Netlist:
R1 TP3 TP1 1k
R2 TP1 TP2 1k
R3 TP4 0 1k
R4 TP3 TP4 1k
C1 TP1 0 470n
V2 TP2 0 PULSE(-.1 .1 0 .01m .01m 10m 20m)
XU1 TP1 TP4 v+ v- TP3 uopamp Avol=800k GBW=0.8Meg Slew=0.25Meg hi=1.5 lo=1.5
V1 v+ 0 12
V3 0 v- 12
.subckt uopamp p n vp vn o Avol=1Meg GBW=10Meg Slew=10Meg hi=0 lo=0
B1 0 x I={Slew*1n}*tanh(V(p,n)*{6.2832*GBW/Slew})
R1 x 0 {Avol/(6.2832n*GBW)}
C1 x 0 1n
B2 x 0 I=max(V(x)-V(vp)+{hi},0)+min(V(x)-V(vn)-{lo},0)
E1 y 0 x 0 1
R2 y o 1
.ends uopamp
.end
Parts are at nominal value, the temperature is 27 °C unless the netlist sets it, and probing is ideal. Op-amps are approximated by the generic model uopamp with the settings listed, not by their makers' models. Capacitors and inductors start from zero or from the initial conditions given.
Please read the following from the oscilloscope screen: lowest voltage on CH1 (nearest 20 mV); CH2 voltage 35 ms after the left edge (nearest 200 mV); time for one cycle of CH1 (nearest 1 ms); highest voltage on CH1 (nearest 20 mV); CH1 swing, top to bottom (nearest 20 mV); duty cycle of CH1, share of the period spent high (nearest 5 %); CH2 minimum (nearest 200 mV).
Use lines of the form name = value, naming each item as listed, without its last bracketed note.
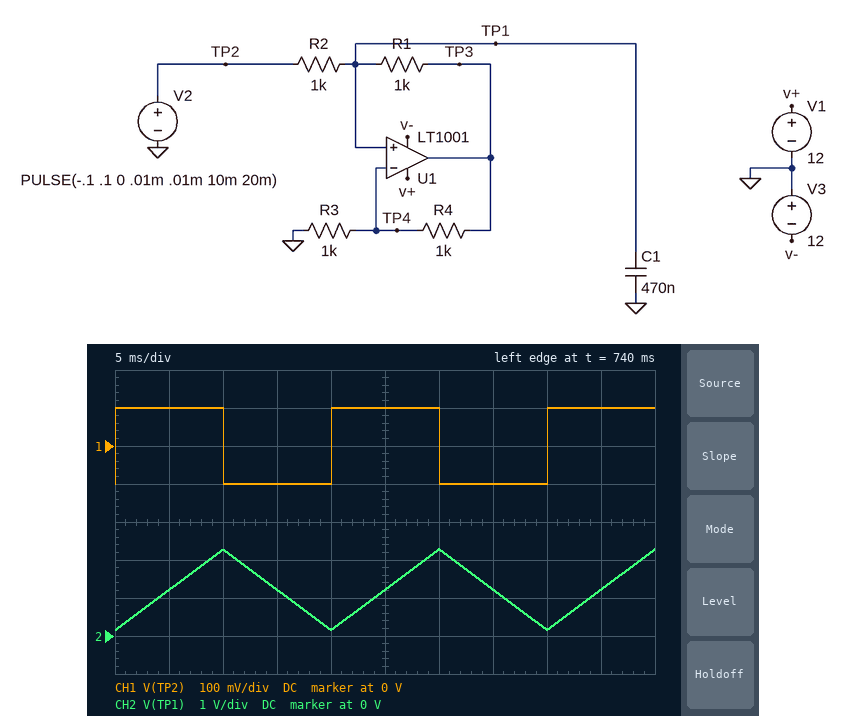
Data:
lowest voltage on CH1 = -100 mV
CH2 voltage 35 ms after the left edge = 1.2 V
time for one cycle of CH1 = 20 ms
highest voltage on CH1 = 100 mV
CH1 swing, top to bottom = 200 mV
duty cycle of CH1, share of the period spent high = 50 %
CH2 minimum = 200 mV
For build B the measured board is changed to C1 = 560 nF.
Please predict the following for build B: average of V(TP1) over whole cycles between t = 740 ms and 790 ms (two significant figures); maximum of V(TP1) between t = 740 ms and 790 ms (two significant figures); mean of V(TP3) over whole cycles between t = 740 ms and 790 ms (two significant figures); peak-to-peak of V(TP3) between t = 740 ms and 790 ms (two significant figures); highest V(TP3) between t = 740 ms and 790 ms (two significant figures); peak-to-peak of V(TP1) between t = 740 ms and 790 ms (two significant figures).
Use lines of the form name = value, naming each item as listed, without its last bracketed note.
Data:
average of V(TP1) over whole cycles between t = 740 ms and 790 ms = 1.0 V
maximum of V(TP1) between t = 740 ms and 790 ms = 1.9 V
mean of V(TP3) over whole cycles between t = 740 ms and 790 ms = 2.0 V
peak-to-peak of V(TP3) between t = 740 ms and 790 ms = 3.6 V
highest V(TP3) between t = 740 ms and 790 ms = 3.8 V
peak-to-peak of V(TP1) between t = 740 ms and 790 ms = 1.8 V
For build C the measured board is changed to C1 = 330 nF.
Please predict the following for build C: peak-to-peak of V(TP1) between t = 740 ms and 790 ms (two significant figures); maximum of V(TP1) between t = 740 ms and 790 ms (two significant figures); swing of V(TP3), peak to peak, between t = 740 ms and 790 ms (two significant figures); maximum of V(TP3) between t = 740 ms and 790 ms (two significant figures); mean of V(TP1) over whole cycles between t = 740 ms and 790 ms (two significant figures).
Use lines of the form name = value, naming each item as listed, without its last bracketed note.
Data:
peak-to-peak of V(TP1) between t = 740 ms and 790 ms = 3.0 V
maximum of V(TP1) between t = 740 ms and 790 ms = 3.2 V
swing of V(TP3), peak to peak, between t = 740 ms and 790 ms = 6.1 V
maximum of V(TP3) between t = 740 ms and 790 ms = 6.5 V
mean of V(TP1) over whole cycles between t = 740 ms and 790 ms = 1.7 V
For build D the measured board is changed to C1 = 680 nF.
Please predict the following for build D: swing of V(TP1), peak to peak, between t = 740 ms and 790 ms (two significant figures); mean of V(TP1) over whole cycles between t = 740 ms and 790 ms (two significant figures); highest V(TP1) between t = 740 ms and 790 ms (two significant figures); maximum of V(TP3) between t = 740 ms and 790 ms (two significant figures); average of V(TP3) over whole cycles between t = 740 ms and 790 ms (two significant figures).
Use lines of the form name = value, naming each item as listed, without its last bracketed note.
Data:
swing of V(TP1), peak to peak, between t = 740 ms and 790 ms = 1.5 V
mean of V(TP1) over whole cycles between t = 740 ms and 790 ms = 840 mV
highest V(TP1) between t = 740 ms and 790 ms = 1.6 V
maximum of V(TP3) between t = 740 ms and 790 ms = 3.2 V
average of V(TP3) over whole cycles between t = 740 ms and 790 ms = 1.7 V
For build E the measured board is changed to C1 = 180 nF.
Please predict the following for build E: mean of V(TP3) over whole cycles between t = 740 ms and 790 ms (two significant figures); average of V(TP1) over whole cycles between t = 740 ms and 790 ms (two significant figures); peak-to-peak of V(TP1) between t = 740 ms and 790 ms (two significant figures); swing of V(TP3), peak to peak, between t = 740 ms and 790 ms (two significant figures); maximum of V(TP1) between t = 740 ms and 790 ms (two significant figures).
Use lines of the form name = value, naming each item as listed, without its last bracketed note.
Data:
mean of V(TP3) over whole cycles between t = 740 ms and 790 ms = 5.0 V
average of V(TP1) over whole cycles between t = 740 ms and 790 ms = 2.5 V
peak-to-peak of V(TP1) between t = 740 ms and 790 ms = 5.5 V
swing of V(TP3), peak to peak, between t = 740 ms and 790 ms = 11 V
maximum of V(TP1) between t = 740 ms and 790 ms = 5.3 V
